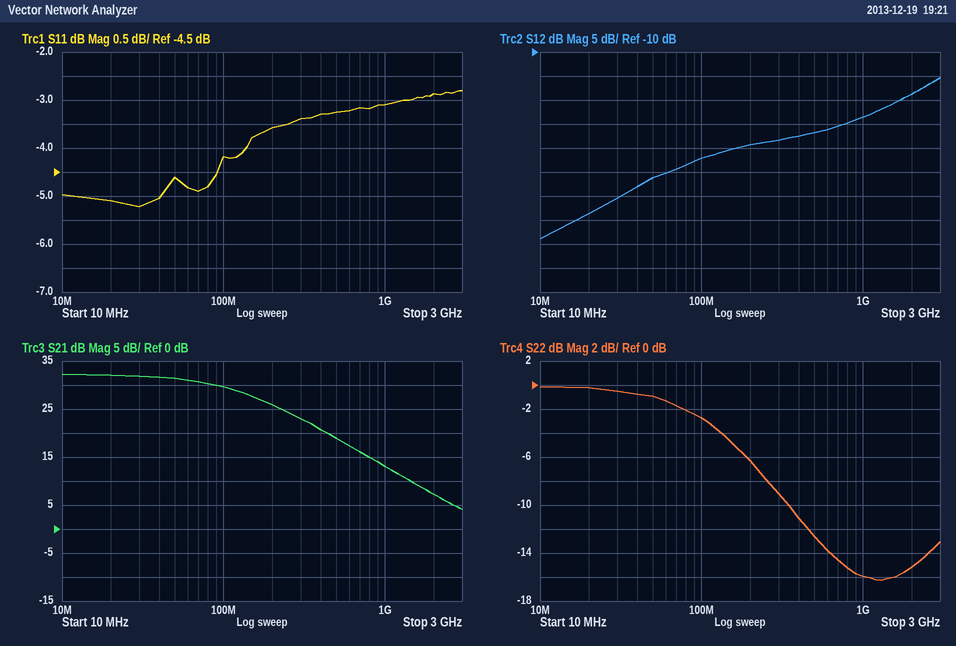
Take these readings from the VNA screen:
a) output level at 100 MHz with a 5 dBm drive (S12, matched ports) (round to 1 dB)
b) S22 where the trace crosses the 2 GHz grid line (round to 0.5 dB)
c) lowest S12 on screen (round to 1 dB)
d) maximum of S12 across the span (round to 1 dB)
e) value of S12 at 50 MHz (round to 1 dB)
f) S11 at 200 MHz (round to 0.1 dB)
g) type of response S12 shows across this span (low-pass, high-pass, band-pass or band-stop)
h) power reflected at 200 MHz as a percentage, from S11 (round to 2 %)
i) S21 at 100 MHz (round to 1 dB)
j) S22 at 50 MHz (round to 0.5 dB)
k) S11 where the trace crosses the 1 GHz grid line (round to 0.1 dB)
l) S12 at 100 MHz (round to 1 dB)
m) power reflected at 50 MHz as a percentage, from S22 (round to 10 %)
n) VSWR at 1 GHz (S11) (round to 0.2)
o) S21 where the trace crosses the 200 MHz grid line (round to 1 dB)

-27 dBm
-15.0 dB
-49 dB
-15 dB
-36 dB
-3.6 dB
high-pass
44 %
30 dB
-1.0 dB
-3.1 dB
-32 dB
80 %
5.6
26 dB
